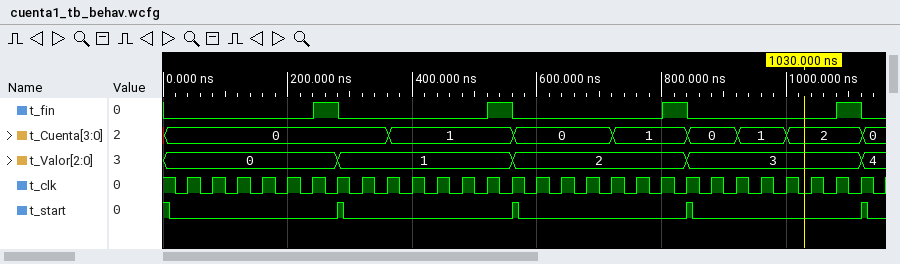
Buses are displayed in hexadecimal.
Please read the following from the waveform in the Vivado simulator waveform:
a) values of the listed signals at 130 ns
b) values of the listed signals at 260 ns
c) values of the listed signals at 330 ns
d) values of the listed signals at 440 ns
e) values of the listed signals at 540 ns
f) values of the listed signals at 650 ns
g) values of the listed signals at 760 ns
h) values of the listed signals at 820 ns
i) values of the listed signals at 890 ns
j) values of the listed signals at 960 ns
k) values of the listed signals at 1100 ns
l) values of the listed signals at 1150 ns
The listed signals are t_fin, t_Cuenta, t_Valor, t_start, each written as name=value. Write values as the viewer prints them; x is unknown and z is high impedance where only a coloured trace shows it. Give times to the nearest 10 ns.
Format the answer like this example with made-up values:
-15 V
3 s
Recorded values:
t_fin=0, t_Cuenta=0, t_Valor=0, t_start=0
t_fin=1, t_Cuenta=0, t_Valor=0, t_start=0
t_fin=0, t_Cuenta=0, t_Valor=1, t_start=0
t_fin=0, t_Cuenta=1, t_Valor=1, t_start=0
t_fin=1, t_Cuenta=1, t_Valor=1, t_start=0
t_fin=0, t_Cuenta=0, t_Valor=2, t_start=0
t_fin=0, t_Cuenta=1, t_Valor=2, t_start=0
t_fin=1, t_Cuenta=1, t_Valor=2, t_start=0
t_fin=0, t_Cuenta=0, t_Valor=3, t_start=0
t_fin=0, t_Cuenta=1, t_Valor=3, t_start=0
t_fin=1, t_Cuenta=2, t_Valor=3, t_start=0
t_fin=0, t_Cuenta=0, t_Valor=4, t_start=0
